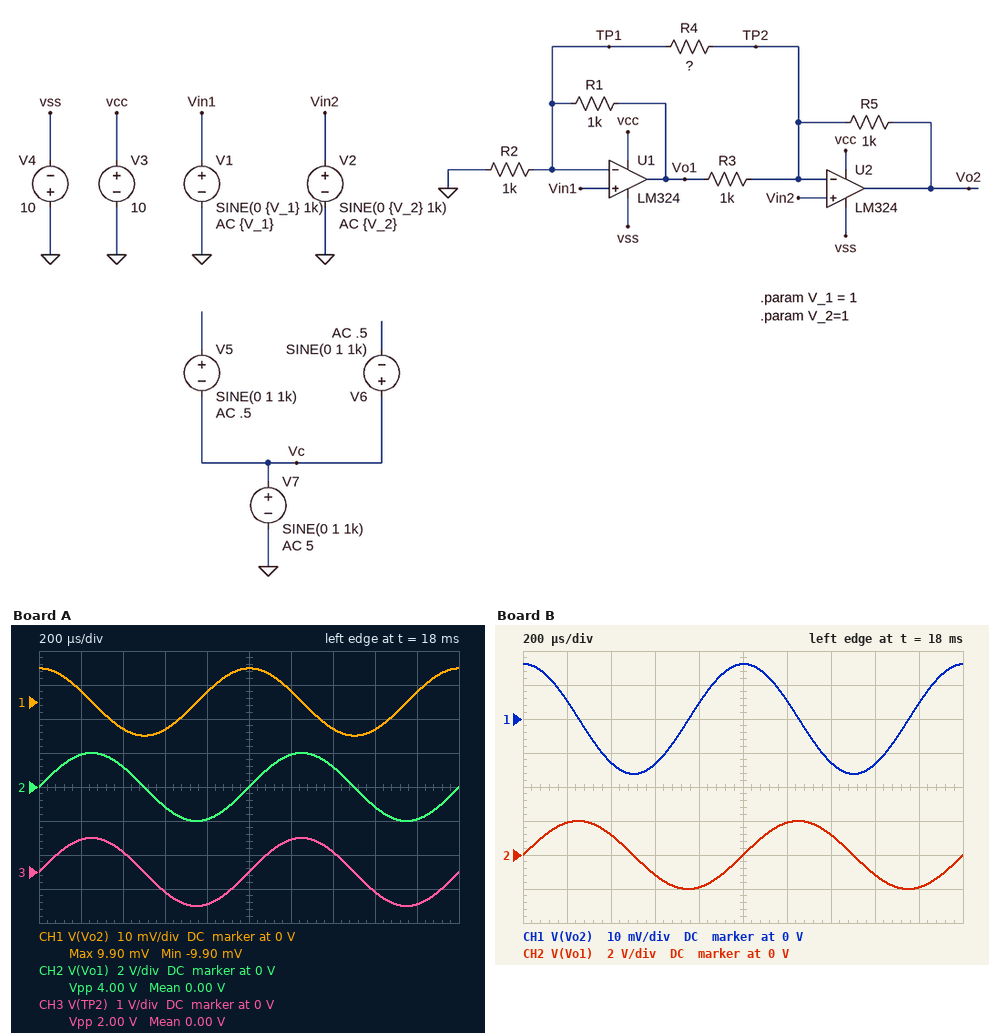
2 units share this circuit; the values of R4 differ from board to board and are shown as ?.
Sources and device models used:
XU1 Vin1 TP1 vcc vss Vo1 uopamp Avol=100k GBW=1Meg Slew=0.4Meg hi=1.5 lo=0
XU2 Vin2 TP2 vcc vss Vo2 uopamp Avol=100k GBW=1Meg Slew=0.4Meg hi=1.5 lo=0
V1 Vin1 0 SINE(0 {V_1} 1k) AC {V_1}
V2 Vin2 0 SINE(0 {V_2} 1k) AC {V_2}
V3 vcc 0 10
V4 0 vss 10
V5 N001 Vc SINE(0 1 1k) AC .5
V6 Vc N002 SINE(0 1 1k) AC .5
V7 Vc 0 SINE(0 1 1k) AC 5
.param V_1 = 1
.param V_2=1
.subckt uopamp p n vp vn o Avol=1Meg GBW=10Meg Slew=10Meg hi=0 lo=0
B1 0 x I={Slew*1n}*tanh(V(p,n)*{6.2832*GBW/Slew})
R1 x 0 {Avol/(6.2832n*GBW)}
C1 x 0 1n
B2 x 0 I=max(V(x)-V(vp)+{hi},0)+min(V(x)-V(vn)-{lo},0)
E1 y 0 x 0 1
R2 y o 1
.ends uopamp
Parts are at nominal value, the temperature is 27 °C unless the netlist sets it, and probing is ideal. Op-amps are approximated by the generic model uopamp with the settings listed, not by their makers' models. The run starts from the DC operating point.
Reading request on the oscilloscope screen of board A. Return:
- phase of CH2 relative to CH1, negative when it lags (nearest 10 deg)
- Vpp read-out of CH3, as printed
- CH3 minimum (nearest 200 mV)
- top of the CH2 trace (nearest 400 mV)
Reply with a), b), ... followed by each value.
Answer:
a) -90 deg
b) 2.00 V
c) -1.0 V
d) 2.0 V
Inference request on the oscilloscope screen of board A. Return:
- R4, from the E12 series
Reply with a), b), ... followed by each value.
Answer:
a) 680 Ω
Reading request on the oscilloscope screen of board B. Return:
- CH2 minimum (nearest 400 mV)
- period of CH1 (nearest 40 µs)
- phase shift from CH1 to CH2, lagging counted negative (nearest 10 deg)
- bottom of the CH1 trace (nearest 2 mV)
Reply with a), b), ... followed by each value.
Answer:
a) -2.0 V
b) 1.00 ms
c) -90 deg
d) -16 mV
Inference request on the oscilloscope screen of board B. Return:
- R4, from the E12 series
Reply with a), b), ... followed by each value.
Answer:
a) 330 Ω
